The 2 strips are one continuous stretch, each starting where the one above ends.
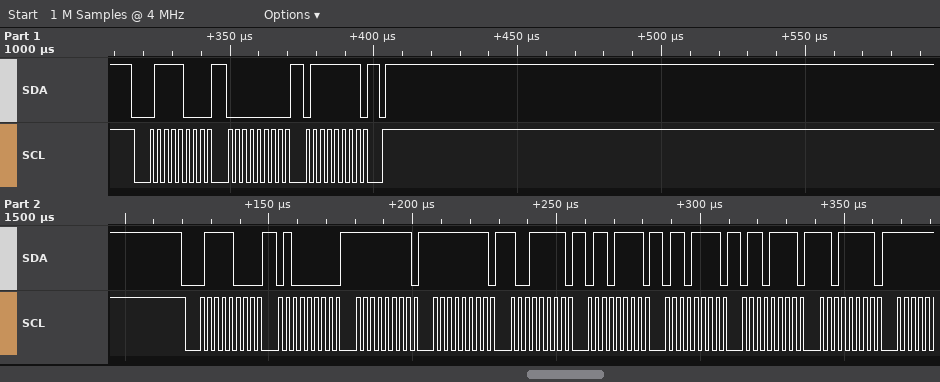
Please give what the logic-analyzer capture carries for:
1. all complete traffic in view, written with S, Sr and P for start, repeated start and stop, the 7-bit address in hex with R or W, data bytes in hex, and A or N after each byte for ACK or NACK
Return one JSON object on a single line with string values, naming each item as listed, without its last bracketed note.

{"all complete traffic in view, written with S, Sr and P for start, repeated start and stop, the 7-bit address in hex with R or W, data bytes in hex, and A or N after each byte for ACK or NACK": "S 3CW A 00 A 7F A P S 3CW A 40 A FF A FF A 9F A 6F A 6F A 6F A DF A"}
